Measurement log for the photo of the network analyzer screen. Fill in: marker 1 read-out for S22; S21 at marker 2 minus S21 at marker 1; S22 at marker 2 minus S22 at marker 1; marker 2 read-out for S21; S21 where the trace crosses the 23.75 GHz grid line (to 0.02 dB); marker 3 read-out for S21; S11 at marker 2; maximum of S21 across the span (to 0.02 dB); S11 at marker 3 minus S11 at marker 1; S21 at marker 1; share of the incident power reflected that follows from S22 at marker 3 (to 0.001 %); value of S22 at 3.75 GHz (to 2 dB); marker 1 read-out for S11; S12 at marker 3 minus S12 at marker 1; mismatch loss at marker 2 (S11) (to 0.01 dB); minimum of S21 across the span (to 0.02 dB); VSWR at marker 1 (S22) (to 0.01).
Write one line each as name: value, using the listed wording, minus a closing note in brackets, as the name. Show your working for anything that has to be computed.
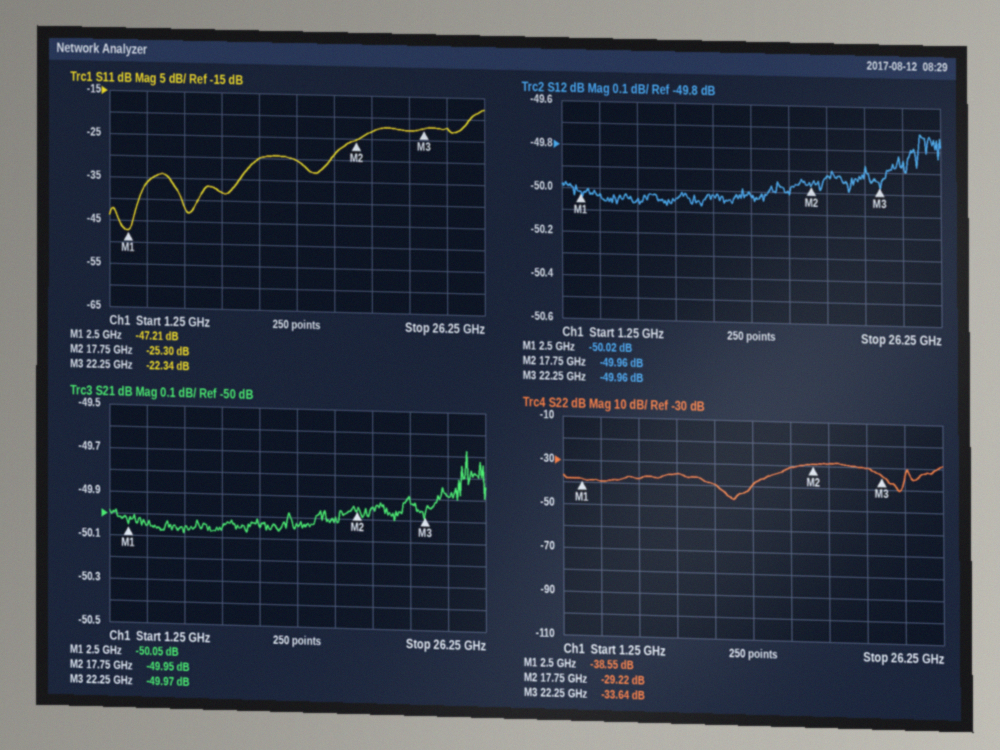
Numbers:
marker 1 read-out for S22: -38.55 dB
S21 at marker 2 minus S21 at marker 1: -49.95 − (-50.05) = 0.10 dB
S22 at marker 2 minus S22 at marker 1: -29.22 − (-38.55) = 9.33 dB
marker 2 read-out for S21: -49.95 dB
S21 where the trace crosses the 23.75 GHz grid line: -49.88 dB
marker 3 read-out for S21: -49.97 dB
S11 at marker 2: -25.30 dB
maximum of S21 across the span: -49.68 dB
S11 at marker 3 minus S11 at marker 1: -22.34 − (-47.21) = 24.87 dB
S21 at marker 1: -50.05 dB
share of the incident power reflected that follows from S22 at marker 3: 10^(-33.64/10) ≈ 0.043 %
value of S22 at 3.75 GHz: -40 dB
marker 1 read-out for S11: -47.21 dB
S12 at marker 3 minus S12 at marker 1: -49.96 − (-50.02) = 0.06 dB
mismatch loss at marker 2 (S11): −10 log10(1 − 10^(-25.3/10)) ≈ 0.01 dB
minimum of S21 across the span: -50.08 dB
VSWR at marker 1 (S22): (1 + 0.0118)/(1 − 0.0118) ≈ 1.02
